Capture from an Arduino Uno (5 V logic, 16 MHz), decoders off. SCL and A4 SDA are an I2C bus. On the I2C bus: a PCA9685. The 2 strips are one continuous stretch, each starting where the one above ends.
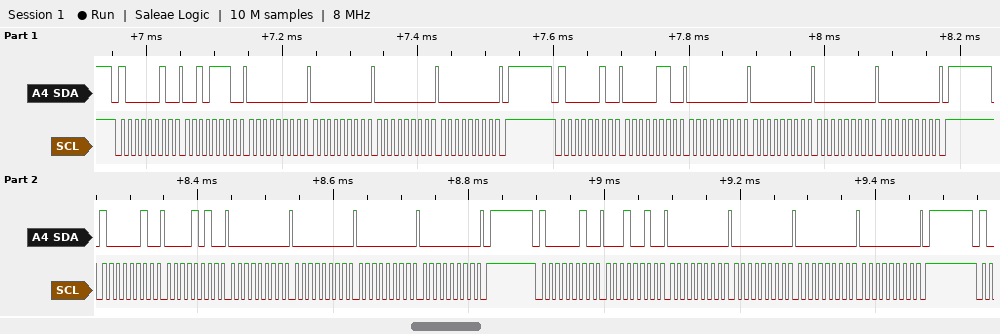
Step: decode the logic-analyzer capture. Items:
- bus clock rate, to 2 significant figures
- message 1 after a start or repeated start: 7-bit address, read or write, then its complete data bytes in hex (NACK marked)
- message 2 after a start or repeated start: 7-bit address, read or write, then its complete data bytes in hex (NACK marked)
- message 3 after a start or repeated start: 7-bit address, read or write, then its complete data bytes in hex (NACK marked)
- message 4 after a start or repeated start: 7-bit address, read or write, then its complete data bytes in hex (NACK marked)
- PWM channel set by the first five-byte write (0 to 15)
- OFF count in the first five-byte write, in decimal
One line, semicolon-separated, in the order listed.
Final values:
100 kHz; 0x41 write: 2E 00 00 00 00; 0x41 write: 06 00 00 00 00; 0x41 write: 0A 00 00 00 00; 0x41 write: 12 00 00 00 00; 10; 0
